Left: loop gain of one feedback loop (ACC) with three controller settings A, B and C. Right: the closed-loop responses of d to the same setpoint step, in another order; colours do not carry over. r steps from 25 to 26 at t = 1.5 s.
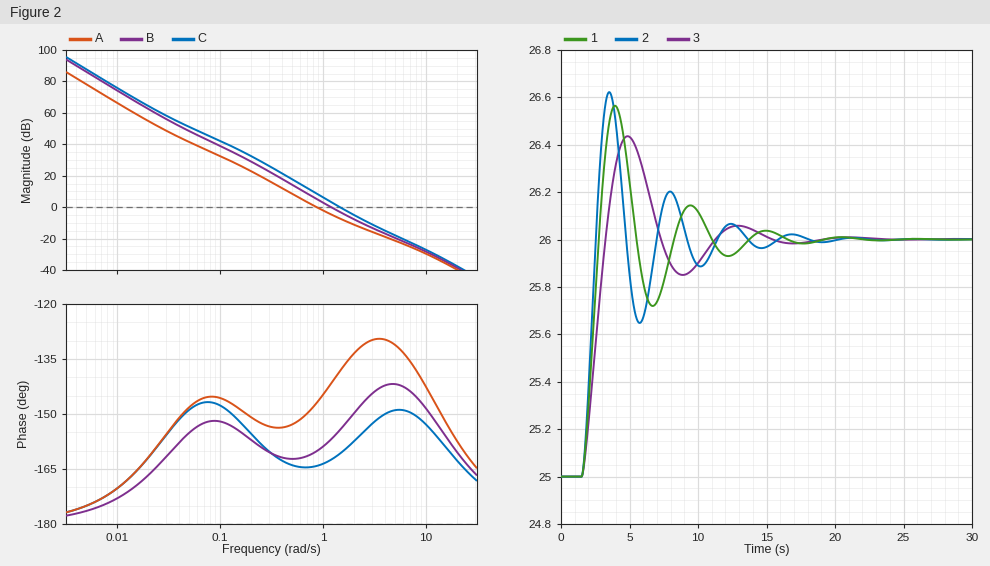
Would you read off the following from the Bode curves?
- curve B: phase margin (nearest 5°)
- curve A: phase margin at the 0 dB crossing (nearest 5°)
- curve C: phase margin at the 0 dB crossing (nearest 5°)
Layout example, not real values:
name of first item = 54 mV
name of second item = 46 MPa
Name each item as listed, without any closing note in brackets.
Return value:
curve B: phase margin = 25°
curve A: phase margin at the 0 dB crossing = 35°
curve C: phase margin at the 0 dB crossing = 20°
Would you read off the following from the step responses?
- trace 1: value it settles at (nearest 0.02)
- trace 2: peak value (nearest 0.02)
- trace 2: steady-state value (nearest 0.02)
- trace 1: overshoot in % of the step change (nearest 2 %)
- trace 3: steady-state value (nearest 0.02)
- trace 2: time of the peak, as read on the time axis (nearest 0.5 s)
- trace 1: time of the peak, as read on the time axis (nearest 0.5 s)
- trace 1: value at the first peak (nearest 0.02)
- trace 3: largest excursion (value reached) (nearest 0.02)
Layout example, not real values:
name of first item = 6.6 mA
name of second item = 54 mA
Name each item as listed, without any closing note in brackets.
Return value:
trace 1: value it settles at = 26.00
trace 2: peak value = 26.62
trace 2: steady-state value = 26.00
trace 1: overshoot in % of the step change = 56 %
trace 3: steady-state value = 26.00
trace 2: time of the peak, as read on the time axis = 3.5 s
trace 1: time of the peak, as read on the time axis = 4.0 s
trace 1: value at the first peak = 26.56
trace 3: largest excursion (value reached) = 26.44
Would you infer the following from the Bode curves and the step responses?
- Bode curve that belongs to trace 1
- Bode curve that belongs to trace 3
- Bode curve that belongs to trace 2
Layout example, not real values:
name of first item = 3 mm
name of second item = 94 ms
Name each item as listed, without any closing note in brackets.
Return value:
Bode curve that belongs to trace 1 = B
Bode curve that belongs to trace 3 = A
Bode curve that belongs to trace 2 = C
